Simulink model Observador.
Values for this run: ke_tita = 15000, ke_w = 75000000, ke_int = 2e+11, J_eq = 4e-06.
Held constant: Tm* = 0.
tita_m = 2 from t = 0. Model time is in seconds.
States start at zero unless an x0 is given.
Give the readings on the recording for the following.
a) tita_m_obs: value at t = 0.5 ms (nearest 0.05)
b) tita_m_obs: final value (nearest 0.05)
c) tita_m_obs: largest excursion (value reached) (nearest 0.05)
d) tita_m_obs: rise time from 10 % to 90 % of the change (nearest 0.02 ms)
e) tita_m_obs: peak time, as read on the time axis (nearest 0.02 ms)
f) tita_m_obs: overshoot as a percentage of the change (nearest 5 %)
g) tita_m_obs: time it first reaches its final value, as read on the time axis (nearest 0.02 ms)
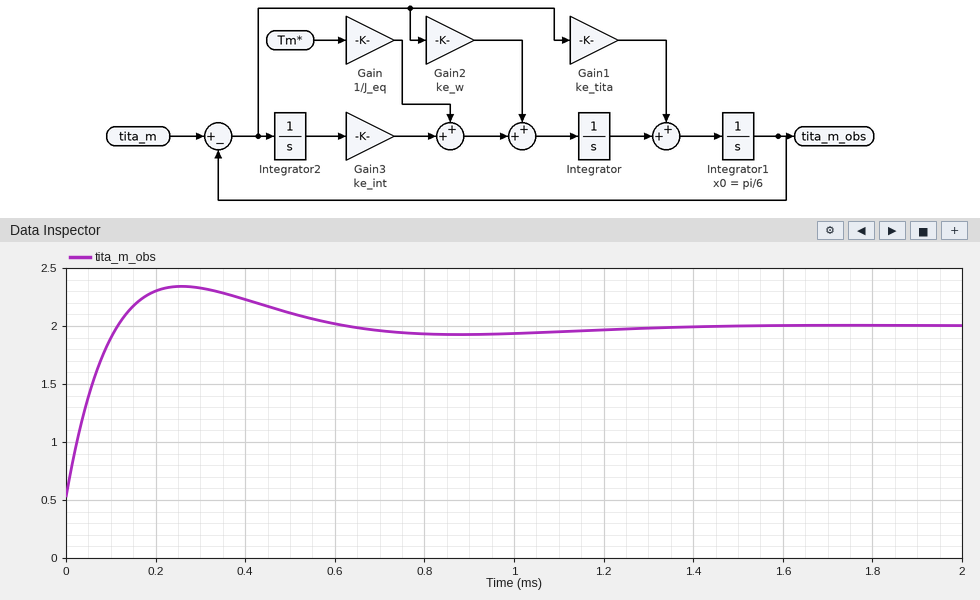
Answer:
2.10
2.00
2.35
0.08 ms
0.26 ms
25 %
0.12 ms
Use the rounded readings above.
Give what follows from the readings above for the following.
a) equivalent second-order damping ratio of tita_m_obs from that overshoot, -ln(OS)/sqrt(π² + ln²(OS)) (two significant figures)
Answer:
0.40
